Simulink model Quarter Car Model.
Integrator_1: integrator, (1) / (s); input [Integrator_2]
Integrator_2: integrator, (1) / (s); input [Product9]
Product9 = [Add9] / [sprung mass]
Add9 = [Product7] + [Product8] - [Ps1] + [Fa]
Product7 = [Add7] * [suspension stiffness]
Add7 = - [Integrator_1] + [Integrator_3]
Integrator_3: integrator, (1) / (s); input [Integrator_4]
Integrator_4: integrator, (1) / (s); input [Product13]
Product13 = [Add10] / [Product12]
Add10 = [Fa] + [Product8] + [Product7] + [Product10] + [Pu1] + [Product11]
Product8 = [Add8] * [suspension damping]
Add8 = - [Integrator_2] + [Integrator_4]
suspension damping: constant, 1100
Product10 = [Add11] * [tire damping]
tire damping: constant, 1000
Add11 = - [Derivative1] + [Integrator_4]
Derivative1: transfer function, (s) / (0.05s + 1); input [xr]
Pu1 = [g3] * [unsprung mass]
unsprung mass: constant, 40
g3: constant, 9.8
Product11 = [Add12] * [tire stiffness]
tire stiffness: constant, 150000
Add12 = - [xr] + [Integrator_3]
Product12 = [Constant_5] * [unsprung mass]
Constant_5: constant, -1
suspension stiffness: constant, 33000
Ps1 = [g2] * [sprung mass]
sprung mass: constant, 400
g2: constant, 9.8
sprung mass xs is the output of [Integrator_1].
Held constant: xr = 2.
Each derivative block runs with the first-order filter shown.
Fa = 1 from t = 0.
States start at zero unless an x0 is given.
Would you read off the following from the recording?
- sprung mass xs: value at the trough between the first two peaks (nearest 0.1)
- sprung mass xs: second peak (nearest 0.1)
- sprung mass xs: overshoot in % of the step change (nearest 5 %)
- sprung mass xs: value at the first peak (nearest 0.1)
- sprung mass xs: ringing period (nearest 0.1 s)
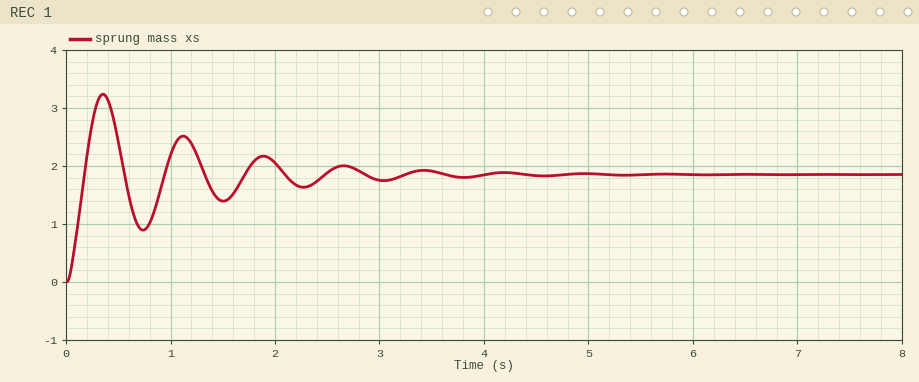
0.9
2.5
75 %
3.2
0.8 s
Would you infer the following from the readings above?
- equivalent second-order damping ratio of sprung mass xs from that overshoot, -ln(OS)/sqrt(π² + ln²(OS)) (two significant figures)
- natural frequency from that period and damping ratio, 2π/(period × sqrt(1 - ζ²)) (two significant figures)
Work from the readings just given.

0.091
7.9 rad/s
